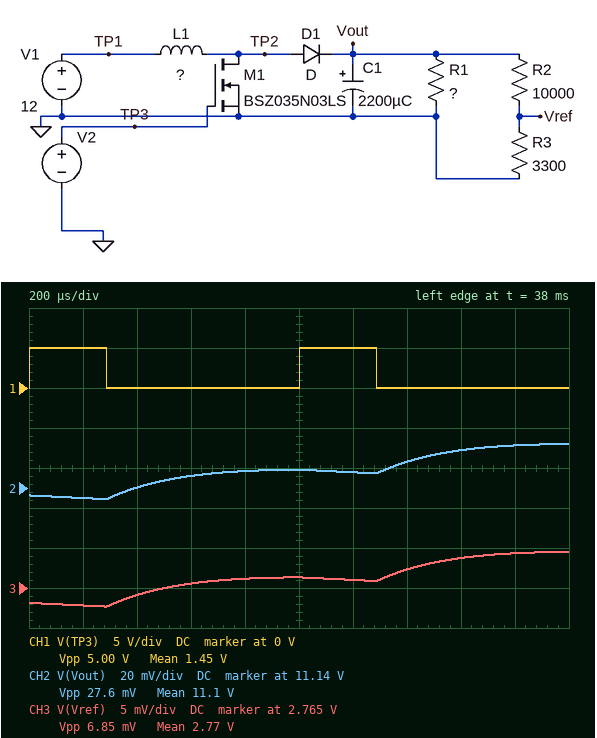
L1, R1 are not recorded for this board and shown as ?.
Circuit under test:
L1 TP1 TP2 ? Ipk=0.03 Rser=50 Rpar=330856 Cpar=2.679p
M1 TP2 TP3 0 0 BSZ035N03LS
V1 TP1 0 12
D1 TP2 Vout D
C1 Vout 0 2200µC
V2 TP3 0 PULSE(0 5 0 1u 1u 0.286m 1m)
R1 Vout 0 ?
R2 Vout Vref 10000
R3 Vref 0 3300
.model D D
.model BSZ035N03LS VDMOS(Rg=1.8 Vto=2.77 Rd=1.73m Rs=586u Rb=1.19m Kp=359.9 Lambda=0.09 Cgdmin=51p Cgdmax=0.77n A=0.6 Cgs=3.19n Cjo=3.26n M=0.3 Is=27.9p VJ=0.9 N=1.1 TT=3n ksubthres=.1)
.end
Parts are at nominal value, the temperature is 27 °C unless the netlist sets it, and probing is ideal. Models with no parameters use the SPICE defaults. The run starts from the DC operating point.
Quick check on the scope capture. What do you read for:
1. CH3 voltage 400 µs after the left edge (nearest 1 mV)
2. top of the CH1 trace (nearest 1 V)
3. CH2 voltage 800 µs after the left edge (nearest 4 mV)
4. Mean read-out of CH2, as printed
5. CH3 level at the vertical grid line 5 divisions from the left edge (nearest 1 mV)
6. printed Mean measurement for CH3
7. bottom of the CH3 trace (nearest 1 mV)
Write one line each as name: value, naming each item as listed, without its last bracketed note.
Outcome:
CH3 voltage 400 µs after the left edge: 2.764 V
top of the CH1 trace: 5 V
CH2 voltage 800 µs after the left edge: 11.148 V
Mean read-out of CH2, as printed: 11.1 V
CH3 level at the vertical grid line 5 divisions from the left edge: 2.766 V
printed Mean measurement for CH3: 2.77 V
bottom of the CH3 trace: 2.763 V
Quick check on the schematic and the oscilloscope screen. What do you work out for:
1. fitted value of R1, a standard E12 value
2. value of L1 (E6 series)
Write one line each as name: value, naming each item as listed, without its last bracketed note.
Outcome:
fitted value of R1, a standard E12 value: 820 Ω
value of L1: 15 mH
